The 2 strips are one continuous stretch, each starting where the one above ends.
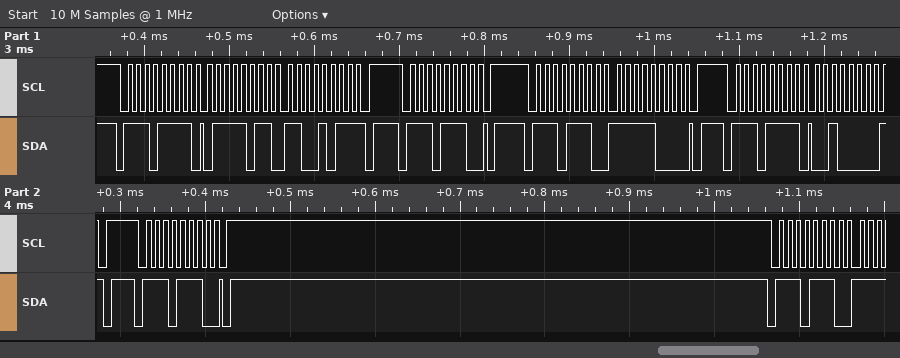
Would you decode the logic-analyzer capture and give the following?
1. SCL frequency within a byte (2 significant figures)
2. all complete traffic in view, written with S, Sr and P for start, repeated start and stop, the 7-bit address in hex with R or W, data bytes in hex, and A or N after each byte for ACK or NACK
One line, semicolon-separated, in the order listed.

100 kHz; S 77R A 7B A CB N P S 77W A P S 77W A F8 A P S 77R A 20 N P S 77W A P S 77W A
